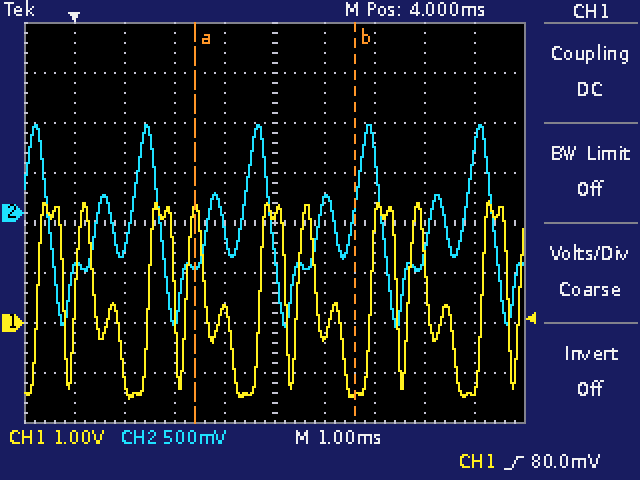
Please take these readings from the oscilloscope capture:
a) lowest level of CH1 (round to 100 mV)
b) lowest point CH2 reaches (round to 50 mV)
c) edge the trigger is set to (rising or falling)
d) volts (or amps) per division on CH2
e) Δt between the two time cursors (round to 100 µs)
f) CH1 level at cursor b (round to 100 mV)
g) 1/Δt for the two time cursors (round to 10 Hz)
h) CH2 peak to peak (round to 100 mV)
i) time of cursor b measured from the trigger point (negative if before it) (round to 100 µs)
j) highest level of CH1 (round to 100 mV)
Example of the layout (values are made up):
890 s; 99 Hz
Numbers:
-1.5 V; -1.15 V; rising; 500 mV; 3.2 ms; -1.4 V; 310 Hz; 2.00 V; +5.6 ms; 2.4 V
